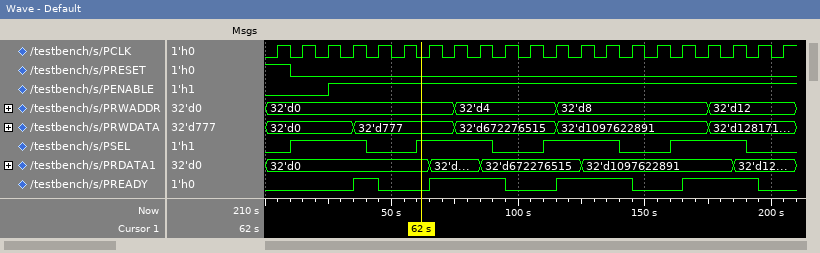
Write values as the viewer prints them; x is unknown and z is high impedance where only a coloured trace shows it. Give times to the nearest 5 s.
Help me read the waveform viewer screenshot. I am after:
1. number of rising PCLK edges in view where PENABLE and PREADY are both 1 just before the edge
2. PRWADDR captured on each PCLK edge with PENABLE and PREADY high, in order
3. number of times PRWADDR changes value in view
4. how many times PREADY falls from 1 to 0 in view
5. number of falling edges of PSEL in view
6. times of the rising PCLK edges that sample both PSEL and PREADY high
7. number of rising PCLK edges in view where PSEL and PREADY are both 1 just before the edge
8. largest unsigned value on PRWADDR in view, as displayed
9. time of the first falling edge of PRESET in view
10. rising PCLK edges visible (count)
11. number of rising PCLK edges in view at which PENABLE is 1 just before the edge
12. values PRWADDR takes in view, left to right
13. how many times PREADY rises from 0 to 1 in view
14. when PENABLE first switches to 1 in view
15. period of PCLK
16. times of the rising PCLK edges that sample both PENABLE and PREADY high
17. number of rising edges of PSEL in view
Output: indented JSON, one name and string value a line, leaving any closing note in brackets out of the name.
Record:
{
  "number of rising PCLK edges in view where PENABLE and PREADY are both 1 just before the edge": "10",
  "PRWADDR captured on each PCLK edge with PENABLE and PREADY high, in order": "32'd0, 32'd0, 32'd4, 32'd4, 32'd8, 32'd8, 32'd8, 32'd8, 32'd12, 32'd12",
  "number of times PRWADDR changes value in view": "3",
  "how many times PREADY falls from 1 to 0 in view": "4",
  "number of falling edges of PSEL in view": "4",
  "times of the rising PCLK edges that sample both PSEL and PREADY high": "75 s, 85 s, 125 s, 135 s, 175 s, 185 s",
  "number of rising PCLK edges in view where PSEL and PREADY are both 1 just before the edge": "6",
  "largest unsigned value on PRWADDR in view, as displayed": "32'd12",
  "time of the first falling edge of PRESET in view": "10 s",
  "rising PCLK edges visible": "21",
  "number of rising PCLK edges in view at which PENABLE is 1 just before the edge": "18",
  "values PRWADDR takes in view, left to right": "32'd0, 32'd4, 32'd8, 32'd12",
  "how many times PREADY rises from 0 to 1 in view": "4",
  "when PENABLE first switches to 1 in view": "25 s",
  "period of PCLK": "10 s",
  "times of the rising PCLK edges that sample both PENABLE and PREADY high": "45 s, 75 s, 85 s, 95 s, 125 s, 135 s, 145 s, 175 s, 185 s, 195 s",
  "number of rising edges of PSEL in view": "4"
}
